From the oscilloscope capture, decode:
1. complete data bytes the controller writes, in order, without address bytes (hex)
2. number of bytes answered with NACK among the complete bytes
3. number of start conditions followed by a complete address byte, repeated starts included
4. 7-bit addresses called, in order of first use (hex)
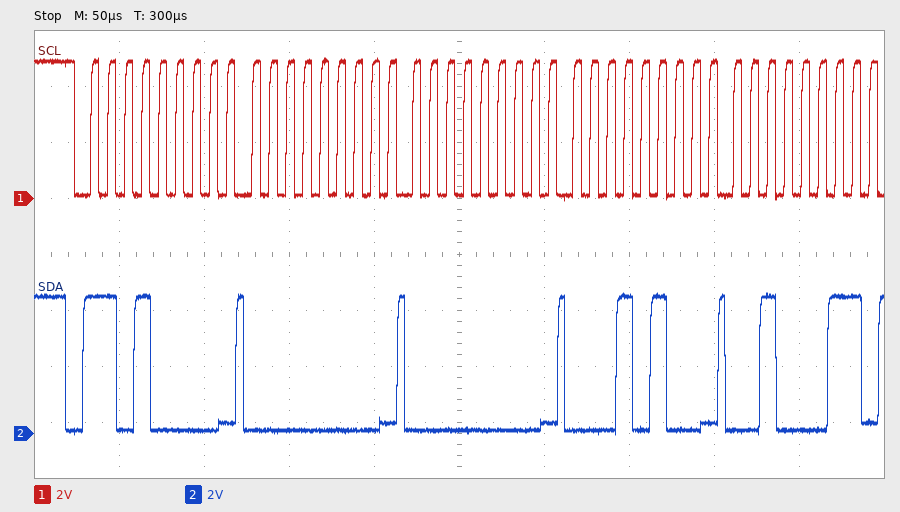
00 00 14 23
0
1
0x68
